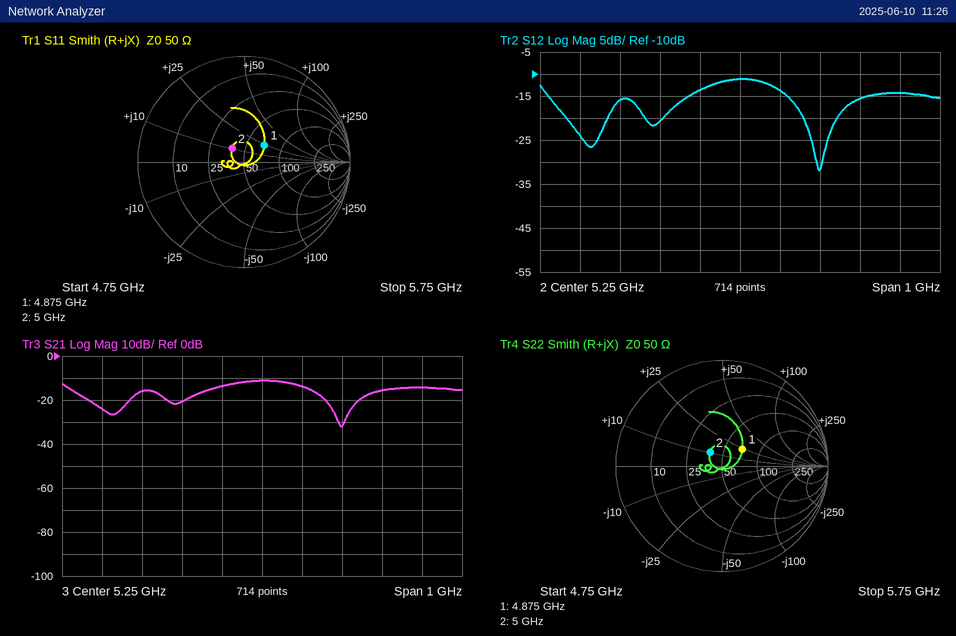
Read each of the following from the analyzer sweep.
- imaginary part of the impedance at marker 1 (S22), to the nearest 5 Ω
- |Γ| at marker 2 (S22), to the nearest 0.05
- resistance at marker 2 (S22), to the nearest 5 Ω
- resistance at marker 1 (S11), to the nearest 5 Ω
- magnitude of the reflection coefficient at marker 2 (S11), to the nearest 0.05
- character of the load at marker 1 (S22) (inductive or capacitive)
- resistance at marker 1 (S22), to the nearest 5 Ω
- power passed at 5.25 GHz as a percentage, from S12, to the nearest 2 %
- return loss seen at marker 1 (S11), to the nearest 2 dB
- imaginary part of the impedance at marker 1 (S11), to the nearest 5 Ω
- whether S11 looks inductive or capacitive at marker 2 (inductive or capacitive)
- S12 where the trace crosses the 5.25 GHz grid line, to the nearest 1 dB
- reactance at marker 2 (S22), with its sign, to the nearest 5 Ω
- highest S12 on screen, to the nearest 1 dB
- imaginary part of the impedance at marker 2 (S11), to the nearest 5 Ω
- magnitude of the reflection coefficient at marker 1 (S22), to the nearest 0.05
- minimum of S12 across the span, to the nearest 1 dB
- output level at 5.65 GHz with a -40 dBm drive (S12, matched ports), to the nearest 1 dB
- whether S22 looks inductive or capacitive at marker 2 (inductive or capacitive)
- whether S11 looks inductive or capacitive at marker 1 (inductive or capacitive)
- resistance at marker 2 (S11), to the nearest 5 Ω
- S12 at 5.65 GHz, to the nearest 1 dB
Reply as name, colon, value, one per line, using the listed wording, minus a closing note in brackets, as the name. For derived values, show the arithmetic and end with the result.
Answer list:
imaginary part of the impedance at marker 1 (S22), to the nearest 5 Ω: +25 Ω
|Γ| at marker 2 (S22), to the nearest 0.05: 0.15
resistance at marker 2 (S22), to the nearest 5 Ω: 40 Ω
resistance at marker 1 (S11), to the nearest 5 Ω: 70 Ω
magnitude of the reflection coefficient at marker 2 (S11), to the nearest 0.05: 0.15
character of the load at marker 1 (S22): inductive
resistance at marker 1 (S22), to the nearest 5 Ω: 70 Ω
power passed at 5.25 GHz as a percentage, from S12, to the nearest 2 %: 10^(-11/10) ≈ 8 %
return loss seen at marker 1 (S11), to the nearest 2 dB: 12 dB
imaginary part of the impedance at marker 1 (S11), to the nearest 5 Ω: +25 Ω
whether S11 looks inductive or capacitive at marker 2: inductive
S12 where the trace crosses the 5.25 GHz grid line, to the nearest 1 dB: -11 dB
reactance at marker 2 (S22), with its sign, to the nearest 5 Ω: +10 Ω
highest S12 on screen, to the nearest 1 dB: -11 dB
imaginary part of the impedance at marker 2 (S11), to the nearest 5 Ω: +10 Ω
magnitude of the reflection coefficient at marker 1 (S22), to the nearest 0.05: 0.25
minimum of S12 across the span, to the nearest 1 dB: -32 dB
output level at 5.65 GHz with a -40 dBm drive (S12, matched ports), to the nearest 1 dB: -40 dBm + (-14 dB) = -54 dBm
whether S22 looks inductive or capacitive at marker 2: inductive
whether S11 looks inductive or capacitive at marker 1: inductive
resistance at marker 2 (S11), to the nearest 5 Ω: 40 Ω
S12 at 5.65 GHz, to the nearest 1 dB: -14 dB
